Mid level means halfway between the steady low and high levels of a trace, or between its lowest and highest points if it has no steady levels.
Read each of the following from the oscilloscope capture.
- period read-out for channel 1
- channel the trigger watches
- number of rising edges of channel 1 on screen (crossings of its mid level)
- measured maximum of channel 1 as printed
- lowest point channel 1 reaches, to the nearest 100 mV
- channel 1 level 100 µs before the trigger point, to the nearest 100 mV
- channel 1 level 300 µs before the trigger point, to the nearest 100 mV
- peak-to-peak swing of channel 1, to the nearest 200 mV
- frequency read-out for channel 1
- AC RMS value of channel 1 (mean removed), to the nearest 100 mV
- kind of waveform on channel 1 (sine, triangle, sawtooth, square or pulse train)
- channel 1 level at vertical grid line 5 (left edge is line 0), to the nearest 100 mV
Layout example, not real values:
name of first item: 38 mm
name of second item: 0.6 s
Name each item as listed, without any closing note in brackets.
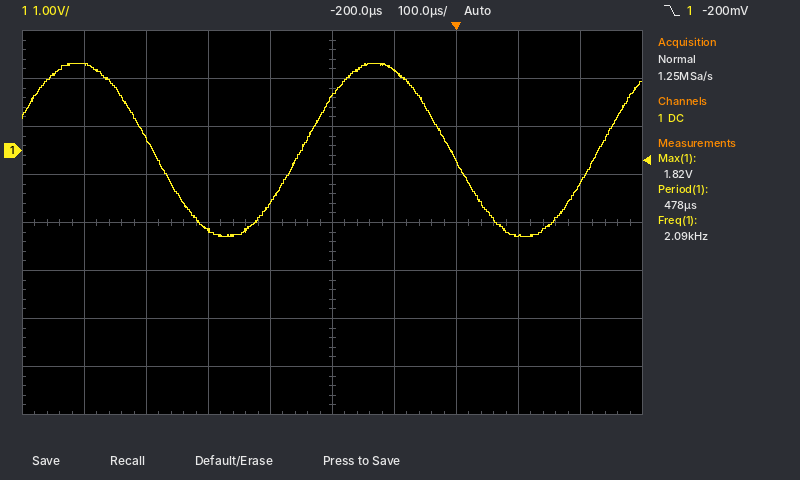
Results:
period read-out for channel 1: 478 µs
channel the trigger watches: channel 1
number of rising edges of channel 1 on screen: 2
measured maximum of channel 1 as printed: 1.82 V
lowest point channel 1 reaches, to the nearest 100 mV: -1.8 V
channel 1 level 100 µs before the trigger point, to the nearest 100 mV: 1.7 V
channel 1 level 300 µs before the trigger point, to the nearest 100 mV: -1.1 V
peak-to-peak swing of channel 1, to the nearest 200 mV: 3.6 V
frequency read-out for channel 1: 2.09 kHz
AC RMS value of channel 1 (mean removed), to the nearest 100 mV: 1.3 V
kind of waveform on channel 1: sine
channel 1 level at vertical grid line 5 (left edge is line 0), to the nearest 100 mV: 1.1 V
